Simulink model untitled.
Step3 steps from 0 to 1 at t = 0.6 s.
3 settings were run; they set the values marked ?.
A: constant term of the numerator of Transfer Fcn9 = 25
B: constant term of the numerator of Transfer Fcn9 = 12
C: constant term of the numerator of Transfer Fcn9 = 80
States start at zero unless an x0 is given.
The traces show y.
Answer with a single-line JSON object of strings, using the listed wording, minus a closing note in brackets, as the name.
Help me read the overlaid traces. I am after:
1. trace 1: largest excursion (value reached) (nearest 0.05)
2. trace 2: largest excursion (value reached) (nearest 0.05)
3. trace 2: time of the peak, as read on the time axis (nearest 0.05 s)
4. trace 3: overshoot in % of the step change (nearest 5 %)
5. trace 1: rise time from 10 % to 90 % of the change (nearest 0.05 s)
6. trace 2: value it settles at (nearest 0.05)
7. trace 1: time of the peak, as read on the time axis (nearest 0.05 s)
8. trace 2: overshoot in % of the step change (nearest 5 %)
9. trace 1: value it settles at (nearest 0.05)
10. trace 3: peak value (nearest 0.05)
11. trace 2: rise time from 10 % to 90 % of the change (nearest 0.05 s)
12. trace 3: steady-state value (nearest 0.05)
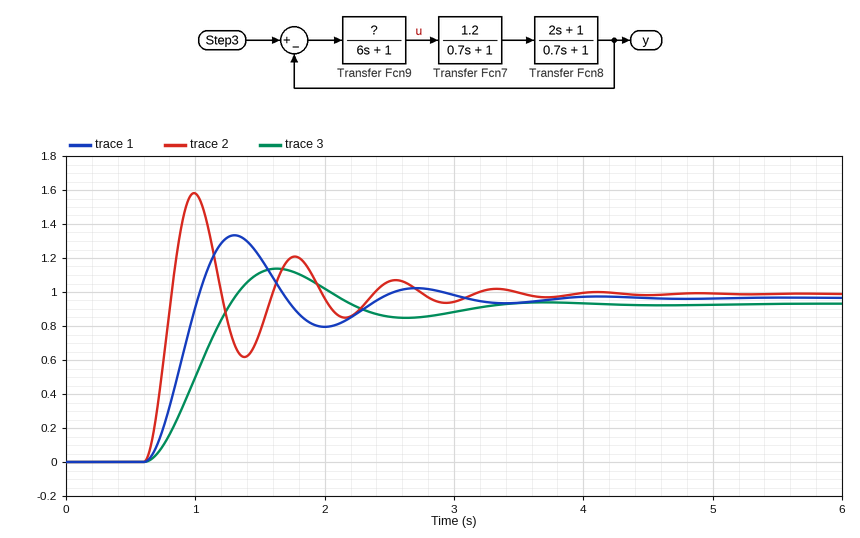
{"trace 1: largest excursion (value reached)": "1.35", "trace 2: largest excursion (value reached)": "1.60", "trace 2: time of the peak, as read on the time axis": "1.00 s", "trace 3: overshoot in % of the step change": "20 %", "trace 1: rise time from 10 % to 90 % of the change": "0.30 s", "trace 2: value it settles at": "1.00", "trace 1: time of the peak, as read on the time axis": "1.30 s", "trace 2: overshoot in % of the step change": "60 %", "trace 1: value it settles at": "0.95", "trace 3: peak value": "1.15", "trace 2: rise time from 10 % to 90 % of the change": "0.15 s", "trace 3: steady-state value": "0.95"}
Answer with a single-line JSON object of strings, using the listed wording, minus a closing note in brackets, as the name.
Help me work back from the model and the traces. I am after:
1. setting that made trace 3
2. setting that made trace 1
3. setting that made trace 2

{"setting that made trace 3": "B", "setting that made trace 1": "A", "setting that made trace 2": "C"}
